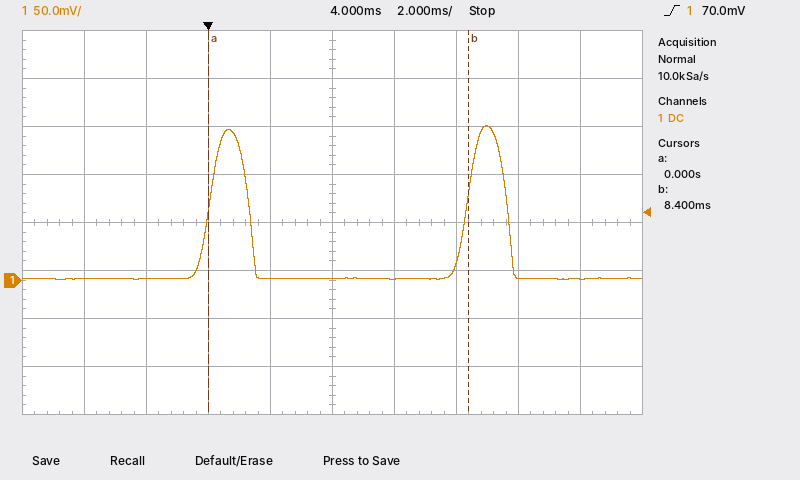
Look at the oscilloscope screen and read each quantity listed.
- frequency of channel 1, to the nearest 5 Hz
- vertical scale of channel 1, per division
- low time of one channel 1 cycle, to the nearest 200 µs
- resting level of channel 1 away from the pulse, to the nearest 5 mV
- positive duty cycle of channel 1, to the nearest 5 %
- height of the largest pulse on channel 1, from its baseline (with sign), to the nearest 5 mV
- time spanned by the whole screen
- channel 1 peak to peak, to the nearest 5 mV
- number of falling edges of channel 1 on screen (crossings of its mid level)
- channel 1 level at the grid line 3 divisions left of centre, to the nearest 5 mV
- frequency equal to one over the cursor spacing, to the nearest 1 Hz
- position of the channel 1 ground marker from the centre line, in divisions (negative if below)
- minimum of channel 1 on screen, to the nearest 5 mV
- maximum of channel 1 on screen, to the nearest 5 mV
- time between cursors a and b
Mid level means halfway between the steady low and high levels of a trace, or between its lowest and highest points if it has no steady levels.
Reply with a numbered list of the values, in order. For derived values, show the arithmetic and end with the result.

1. 120 Hz
2. 50 mV
3. 7.0 ms
4. 0 mV
5. 15 %
6. 160 mV − (0 mV) = +160 mV
7. 20 ms
8. 160 mV − (0 mV) = 160 mV
9. 2
10. 0 mV
11. 1 / 8.4 ms ≈ 119 Hz
12. -1.2 div
13. 0 mV
14. 160 mV
15. 8.4 ms − (0 s) = 8.4 ms
